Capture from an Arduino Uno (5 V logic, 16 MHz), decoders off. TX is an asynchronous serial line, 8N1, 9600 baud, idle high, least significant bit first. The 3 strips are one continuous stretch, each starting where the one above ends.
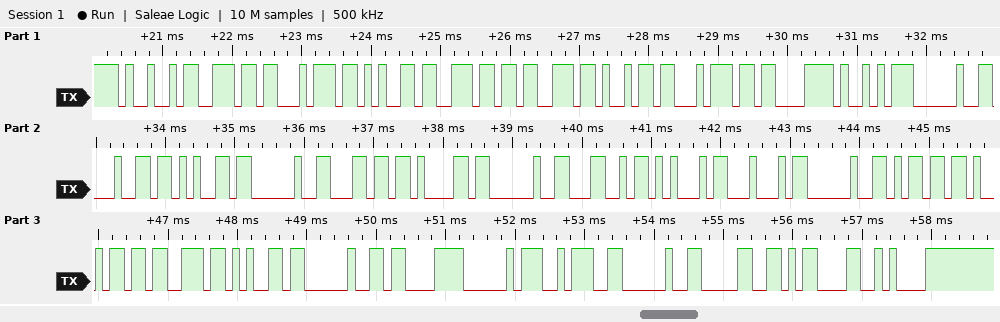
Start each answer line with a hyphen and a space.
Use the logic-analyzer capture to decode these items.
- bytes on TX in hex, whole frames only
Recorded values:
- 49 6E 74 65 6E 73 69 74 C3 A9 20 64 65 20 6C 61 20 4C 45 44 20 6D 69 73 65 20 C3 A0 3A 20 30 0D 0A
